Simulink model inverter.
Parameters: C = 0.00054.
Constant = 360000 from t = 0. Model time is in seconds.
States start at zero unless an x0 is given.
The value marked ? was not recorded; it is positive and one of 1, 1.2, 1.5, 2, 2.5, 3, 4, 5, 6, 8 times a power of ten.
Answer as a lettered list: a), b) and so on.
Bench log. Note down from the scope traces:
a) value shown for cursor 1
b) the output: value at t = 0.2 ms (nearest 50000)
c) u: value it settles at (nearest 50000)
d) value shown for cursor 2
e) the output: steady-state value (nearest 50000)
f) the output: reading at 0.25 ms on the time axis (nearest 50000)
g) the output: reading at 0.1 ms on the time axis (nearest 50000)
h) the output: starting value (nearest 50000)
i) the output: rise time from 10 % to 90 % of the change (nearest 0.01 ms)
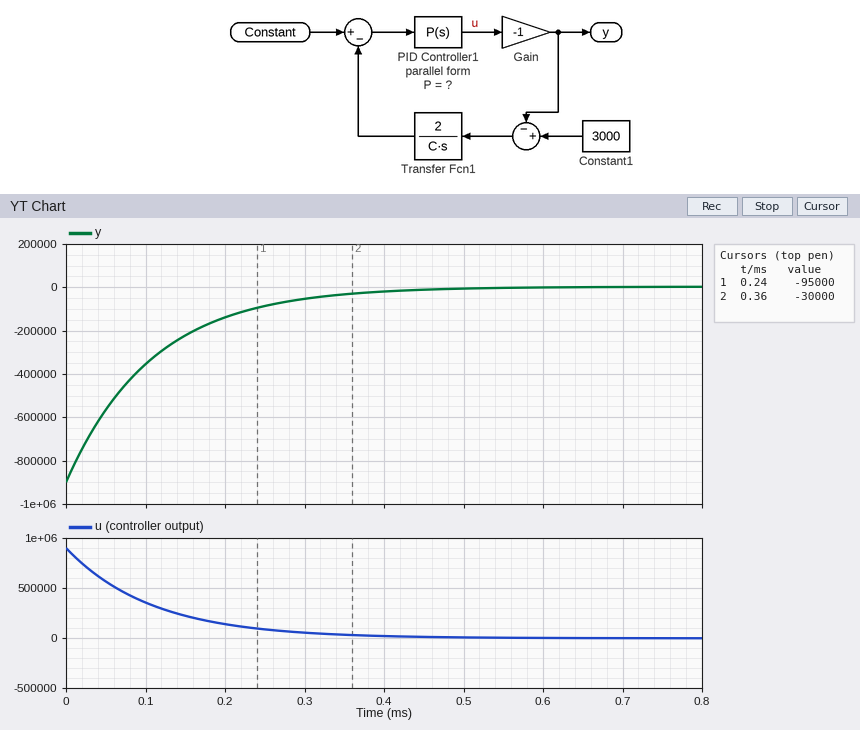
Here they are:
a) -95000
b) -150000
c) 0
d) -30000
e) 0
f) -100000
g) -350000
h) -900000
i) 0.24 ms
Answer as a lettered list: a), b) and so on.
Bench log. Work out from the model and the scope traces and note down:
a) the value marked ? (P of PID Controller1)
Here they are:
a) 2.5
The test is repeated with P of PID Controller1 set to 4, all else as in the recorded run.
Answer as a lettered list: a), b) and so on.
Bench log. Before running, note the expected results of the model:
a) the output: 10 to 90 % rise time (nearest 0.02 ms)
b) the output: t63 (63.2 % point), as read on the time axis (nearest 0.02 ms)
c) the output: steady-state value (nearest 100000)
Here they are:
a) 0.14 ms
b) 0.06 ms
c) 0
